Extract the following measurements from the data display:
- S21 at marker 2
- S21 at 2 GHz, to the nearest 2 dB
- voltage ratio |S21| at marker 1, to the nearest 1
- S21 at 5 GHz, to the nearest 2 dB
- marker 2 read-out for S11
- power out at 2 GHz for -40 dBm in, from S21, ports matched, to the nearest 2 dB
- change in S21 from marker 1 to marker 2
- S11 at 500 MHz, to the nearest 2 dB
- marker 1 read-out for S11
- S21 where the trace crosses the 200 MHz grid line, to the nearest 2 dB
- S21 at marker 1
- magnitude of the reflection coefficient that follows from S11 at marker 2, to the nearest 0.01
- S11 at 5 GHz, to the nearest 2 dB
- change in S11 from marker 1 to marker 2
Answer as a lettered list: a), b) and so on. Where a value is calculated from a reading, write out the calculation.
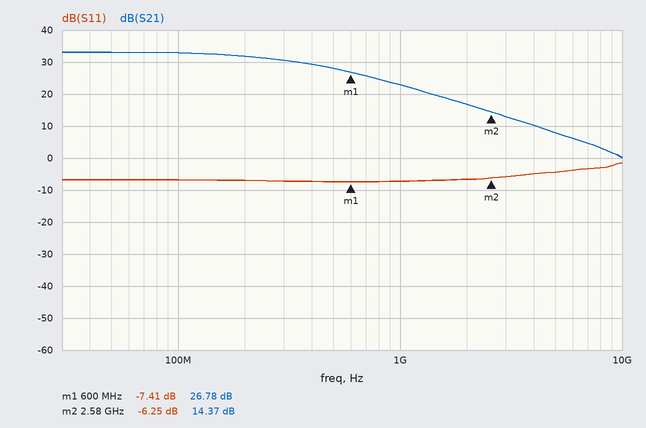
a) 14.37 dB
b) 16 dB
c) 10^(26.78/20) ≈ 22
d) 8 dB
e) -6.25 dB
f) -40 dBm + (16 dB) = -24 dBm
g) 14.37 − (26.78) = -12.41 dB
h) -8 dB
i) -7.41 dB
j) 32 dB
k) 26.78 dB
l) 10^(-6.25/20) ≈ 0.49
m) -4 dB
n) -6.25 − (-7.41) = 1.16 dB
